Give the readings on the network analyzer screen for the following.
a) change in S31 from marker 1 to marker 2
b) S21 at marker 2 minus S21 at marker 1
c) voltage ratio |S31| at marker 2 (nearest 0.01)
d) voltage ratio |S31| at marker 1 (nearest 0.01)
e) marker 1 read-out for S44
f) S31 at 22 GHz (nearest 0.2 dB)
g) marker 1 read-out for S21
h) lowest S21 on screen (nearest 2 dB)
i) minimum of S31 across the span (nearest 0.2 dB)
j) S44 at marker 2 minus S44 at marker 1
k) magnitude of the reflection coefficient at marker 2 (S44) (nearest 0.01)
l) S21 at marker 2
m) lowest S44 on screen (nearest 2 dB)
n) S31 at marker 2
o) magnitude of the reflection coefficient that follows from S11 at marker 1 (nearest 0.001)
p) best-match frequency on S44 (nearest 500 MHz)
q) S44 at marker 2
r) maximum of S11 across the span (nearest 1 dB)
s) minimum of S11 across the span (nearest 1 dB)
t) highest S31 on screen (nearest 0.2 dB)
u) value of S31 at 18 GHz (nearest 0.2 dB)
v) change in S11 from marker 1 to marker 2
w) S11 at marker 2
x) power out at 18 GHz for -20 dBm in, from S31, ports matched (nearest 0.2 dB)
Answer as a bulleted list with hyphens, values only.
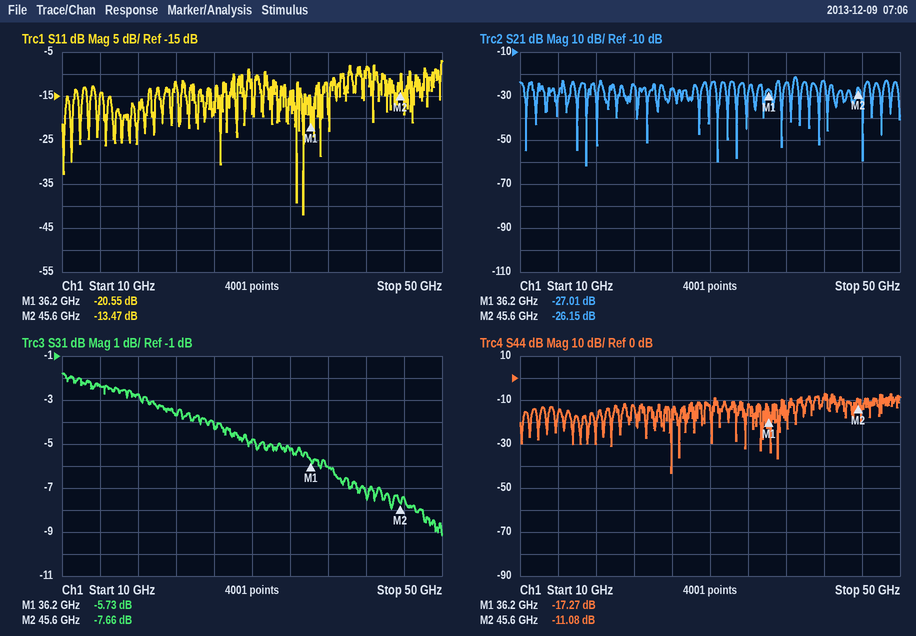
- -1.93 dB
- 0.86 dB
- 0.41
- 0.52
- -17.27 dB
- -3.6 dB
- -27.01 dB
- -62 dB
- -9.2 dB
- 6.19 dB
- 0.28
- -26.15 dB
- -44 dB
- -7.66 dB
- 0.094
- 26.0 GHz
- -11.08 dB
- -7 dB
- -42 dB
- -1.8 dB
- -2.8 dB
- 7.08 dB
- -13.47 dB
- -22.8 dBm
